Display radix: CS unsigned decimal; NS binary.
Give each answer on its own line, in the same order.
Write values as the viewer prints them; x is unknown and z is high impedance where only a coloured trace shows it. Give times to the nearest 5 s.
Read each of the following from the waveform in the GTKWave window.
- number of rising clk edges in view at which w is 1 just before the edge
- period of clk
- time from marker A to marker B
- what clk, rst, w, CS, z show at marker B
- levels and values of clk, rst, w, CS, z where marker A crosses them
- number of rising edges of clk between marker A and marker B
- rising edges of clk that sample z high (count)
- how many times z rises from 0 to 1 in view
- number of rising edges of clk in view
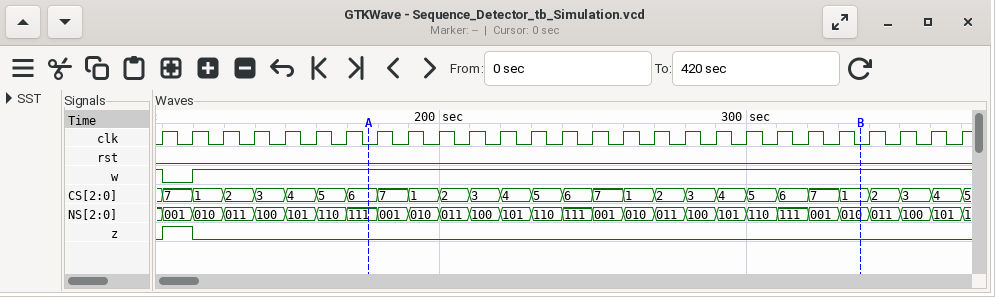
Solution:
26
10 s
160 s
clk=0, rst=0, w=1, CS=1, z=0
clk=0, rst=0, w=1, CS=6, z=0
16
1
1
27
